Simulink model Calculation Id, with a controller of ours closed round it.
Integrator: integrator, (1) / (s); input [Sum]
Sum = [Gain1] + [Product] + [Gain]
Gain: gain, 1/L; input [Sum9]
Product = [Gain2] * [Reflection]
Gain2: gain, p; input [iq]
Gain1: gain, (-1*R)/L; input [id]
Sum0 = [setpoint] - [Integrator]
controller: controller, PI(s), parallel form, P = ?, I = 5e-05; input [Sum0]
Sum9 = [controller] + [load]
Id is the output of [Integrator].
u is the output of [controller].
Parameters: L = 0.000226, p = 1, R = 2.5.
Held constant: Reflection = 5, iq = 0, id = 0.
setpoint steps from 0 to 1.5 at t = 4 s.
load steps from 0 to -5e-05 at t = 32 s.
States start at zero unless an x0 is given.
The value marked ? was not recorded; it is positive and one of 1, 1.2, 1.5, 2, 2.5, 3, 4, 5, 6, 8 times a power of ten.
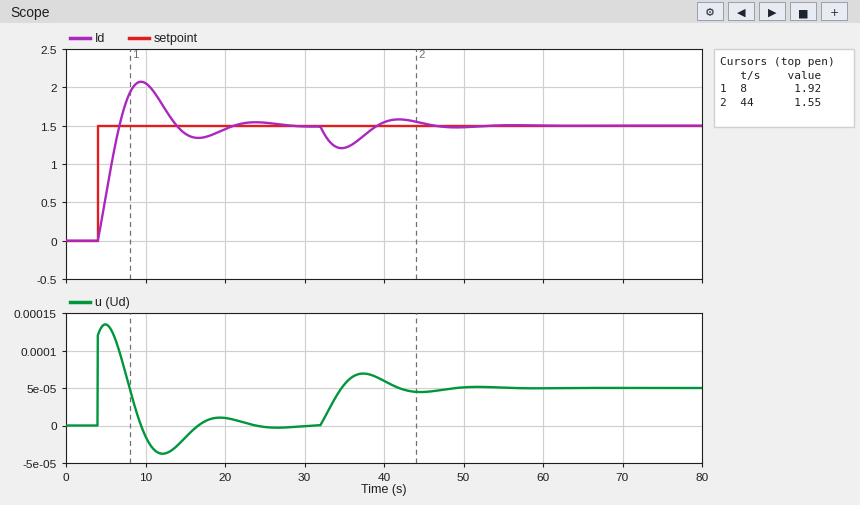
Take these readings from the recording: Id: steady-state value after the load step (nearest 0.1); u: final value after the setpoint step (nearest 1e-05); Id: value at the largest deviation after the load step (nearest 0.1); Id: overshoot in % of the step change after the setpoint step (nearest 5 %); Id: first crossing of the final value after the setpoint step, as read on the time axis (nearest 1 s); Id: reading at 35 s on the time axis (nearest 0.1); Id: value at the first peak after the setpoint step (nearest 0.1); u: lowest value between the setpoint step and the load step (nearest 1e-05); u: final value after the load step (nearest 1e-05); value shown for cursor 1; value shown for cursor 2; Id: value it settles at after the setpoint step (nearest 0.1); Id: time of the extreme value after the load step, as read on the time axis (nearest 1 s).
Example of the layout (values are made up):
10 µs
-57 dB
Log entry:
1.5
0.00000
1.2
40 %
7 s
1.2
2.1
-0.00004
0.00005
1.92
1.55
1.5
35 s
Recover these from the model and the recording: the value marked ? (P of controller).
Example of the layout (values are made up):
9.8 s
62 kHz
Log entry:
8e-05
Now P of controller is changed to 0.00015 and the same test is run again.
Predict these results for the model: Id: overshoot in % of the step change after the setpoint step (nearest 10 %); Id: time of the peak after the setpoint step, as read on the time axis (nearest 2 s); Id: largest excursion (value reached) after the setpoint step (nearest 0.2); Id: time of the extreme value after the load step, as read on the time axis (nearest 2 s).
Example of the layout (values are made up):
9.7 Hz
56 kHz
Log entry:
20 %
8 s
1.8
34 s
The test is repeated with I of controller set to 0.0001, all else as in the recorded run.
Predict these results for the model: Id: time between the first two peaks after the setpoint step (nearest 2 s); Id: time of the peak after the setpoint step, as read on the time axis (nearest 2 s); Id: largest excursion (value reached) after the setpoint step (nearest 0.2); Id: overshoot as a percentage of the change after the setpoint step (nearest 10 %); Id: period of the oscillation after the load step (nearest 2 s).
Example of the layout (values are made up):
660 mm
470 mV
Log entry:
10 s
8 s
2.2
50 %
10 s
